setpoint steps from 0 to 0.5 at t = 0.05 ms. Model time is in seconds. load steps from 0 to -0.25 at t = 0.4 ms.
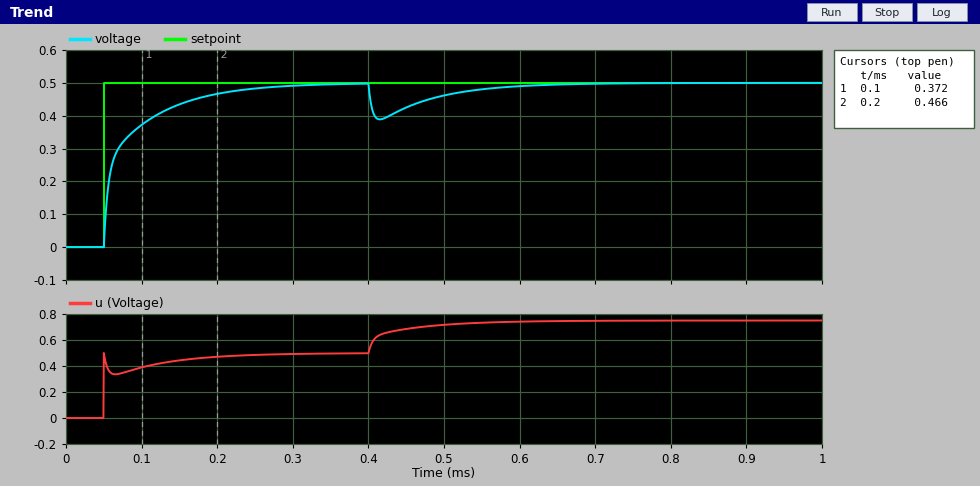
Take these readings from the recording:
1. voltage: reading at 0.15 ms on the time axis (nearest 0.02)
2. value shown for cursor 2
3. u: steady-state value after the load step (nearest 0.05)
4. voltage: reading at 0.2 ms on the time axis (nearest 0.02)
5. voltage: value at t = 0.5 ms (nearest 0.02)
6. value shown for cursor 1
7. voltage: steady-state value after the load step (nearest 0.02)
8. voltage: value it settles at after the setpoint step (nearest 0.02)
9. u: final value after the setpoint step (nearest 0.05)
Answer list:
0.44
0.466
0.75
0.46
0.46
0.372
0.50
0.50
0.50
